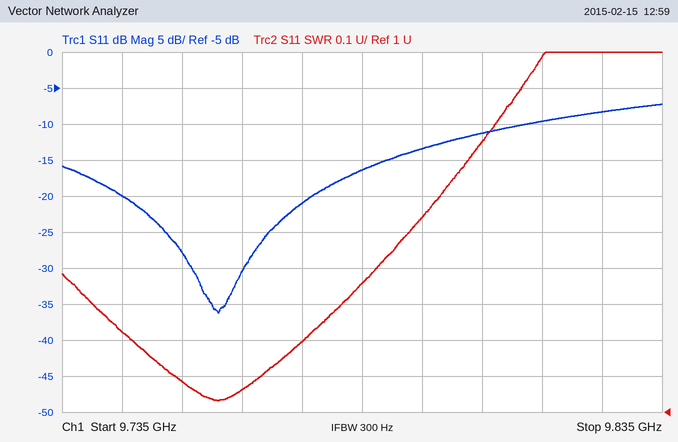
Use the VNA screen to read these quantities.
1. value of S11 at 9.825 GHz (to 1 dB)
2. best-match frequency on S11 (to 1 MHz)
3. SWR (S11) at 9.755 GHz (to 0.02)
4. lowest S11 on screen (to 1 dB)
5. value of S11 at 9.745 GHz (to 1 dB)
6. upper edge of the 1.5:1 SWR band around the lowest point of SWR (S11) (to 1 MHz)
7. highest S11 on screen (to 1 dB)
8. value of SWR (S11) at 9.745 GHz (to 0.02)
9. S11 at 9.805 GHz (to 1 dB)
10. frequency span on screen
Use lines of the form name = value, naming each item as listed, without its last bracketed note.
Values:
value of S11 at 9.825 GHz = -8 dB
best-match frequency on S11 = 9.761 GHz
SWR (S11) at 9.755 GHz = 1.08
lowest S11 on screen = -36 dB
value of S11 at 9.745 GHz = -20 dB
upper edge of the 1.5:1 SWR band around the lowest point of SWR (S11) = 9.793 GHz
highest S11 on screen = -7 dB
value of SWR (S11) at 9.745 GHz = 1.22
S11 at 9.805 GHz = -11 dB
frequency span on screen = 100 MHz
